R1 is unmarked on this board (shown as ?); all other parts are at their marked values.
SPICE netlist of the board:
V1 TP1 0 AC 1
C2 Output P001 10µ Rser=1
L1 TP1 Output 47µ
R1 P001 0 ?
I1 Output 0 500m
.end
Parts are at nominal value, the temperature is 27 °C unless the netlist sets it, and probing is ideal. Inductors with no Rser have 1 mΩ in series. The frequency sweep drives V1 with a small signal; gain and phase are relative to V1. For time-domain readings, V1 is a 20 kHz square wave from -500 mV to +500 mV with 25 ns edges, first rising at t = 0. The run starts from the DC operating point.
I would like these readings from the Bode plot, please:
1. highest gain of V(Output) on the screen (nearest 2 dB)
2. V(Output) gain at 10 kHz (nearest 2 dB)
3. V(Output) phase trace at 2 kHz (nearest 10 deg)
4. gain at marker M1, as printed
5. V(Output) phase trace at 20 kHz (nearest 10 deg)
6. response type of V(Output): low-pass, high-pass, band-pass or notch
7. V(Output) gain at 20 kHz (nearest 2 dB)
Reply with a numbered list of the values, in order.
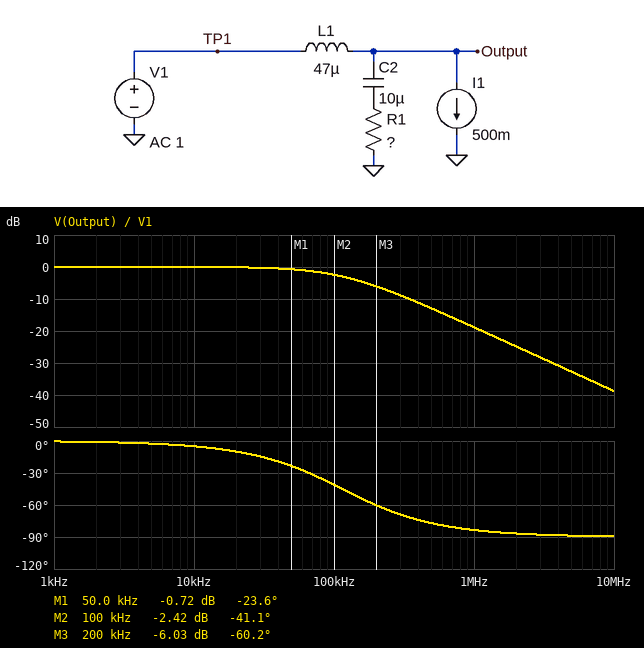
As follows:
1. 0 dB
2. 0 dB
3. 0 deg
4. -0.72 dB
5. -10 deg
6. low-pass
7. 0 dB
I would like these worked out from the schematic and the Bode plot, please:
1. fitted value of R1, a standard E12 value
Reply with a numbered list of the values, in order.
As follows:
1. 33 Ω
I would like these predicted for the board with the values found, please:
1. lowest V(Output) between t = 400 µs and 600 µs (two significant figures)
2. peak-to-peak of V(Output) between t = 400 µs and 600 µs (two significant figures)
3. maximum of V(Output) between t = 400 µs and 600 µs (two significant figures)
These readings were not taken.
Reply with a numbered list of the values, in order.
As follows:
1. -500 mV
2. 1.0 V
3. 500 mV
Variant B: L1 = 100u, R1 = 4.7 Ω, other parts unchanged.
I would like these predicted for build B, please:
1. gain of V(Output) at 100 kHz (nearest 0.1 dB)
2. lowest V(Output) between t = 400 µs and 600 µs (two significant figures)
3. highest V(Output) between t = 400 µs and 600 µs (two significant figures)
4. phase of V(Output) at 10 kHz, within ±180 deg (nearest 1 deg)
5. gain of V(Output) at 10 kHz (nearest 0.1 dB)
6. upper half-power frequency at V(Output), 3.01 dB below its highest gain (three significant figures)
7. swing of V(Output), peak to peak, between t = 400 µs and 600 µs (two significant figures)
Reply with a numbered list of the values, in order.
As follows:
1. -20.9 dB
2. -330 mV
3. 330 mV
4. -55 deg
5. -1.9 dB
6. 9.43 kHz
7. 670 mV
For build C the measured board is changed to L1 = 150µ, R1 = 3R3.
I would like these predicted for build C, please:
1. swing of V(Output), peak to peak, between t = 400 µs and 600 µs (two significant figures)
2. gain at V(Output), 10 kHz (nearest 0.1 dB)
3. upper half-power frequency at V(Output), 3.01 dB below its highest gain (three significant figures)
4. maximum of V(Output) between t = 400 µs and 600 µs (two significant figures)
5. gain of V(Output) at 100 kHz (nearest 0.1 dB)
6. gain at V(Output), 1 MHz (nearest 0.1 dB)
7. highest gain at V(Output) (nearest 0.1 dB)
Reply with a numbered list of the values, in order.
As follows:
1. 370 mV
2. -5.8 dB
3. 5.87 kHz
4. 180 mV
5. -26.8 dB
6. -46.8 dB
7. 2.9 dB
